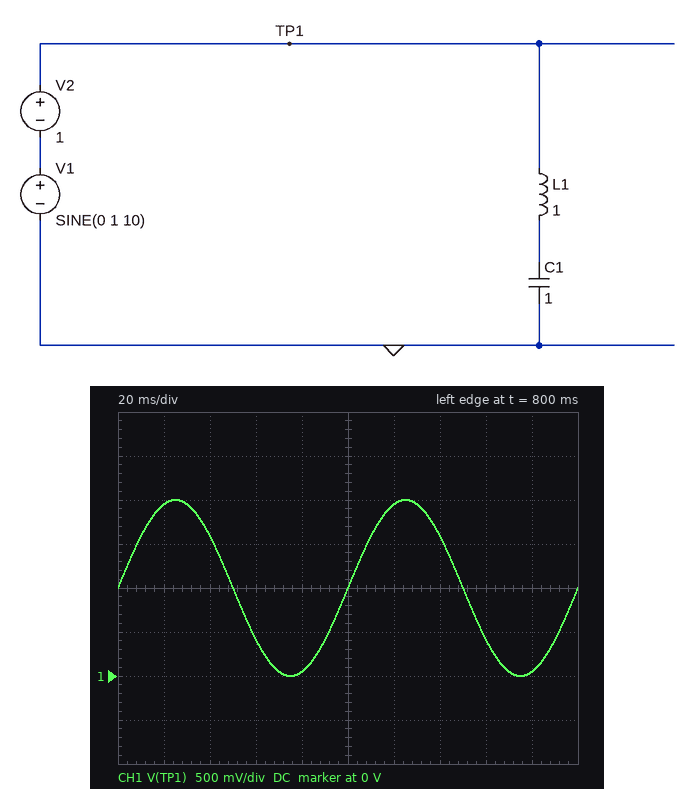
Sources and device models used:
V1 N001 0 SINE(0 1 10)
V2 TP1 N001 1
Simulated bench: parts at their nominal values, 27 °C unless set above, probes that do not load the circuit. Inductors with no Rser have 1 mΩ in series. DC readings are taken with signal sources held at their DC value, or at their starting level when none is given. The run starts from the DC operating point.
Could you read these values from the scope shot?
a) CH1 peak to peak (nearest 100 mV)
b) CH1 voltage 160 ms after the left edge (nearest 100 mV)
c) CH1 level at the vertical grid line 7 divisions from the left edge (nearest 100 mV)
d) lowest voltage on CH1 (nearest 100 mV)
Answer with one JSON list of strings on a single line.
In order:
["2.0 V", "400 mV", "1.6 V", "0 V"]
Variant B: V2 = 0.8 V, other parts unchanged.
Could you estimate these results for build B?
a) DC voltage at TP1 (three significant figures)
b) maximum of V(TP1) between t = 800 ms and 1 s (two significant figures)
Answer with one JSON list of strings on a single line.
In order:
["800 mV", "1.8 V"]
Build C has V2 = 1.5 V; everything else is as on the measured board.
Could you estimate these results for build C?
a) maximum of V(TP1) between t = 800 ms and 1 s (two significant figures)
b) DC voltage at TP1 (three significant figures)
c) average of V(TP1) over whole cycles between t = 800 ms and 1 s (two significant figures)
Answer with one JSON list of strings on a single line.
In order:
["2.5 V", "1.50 V", "1.5 V"]
